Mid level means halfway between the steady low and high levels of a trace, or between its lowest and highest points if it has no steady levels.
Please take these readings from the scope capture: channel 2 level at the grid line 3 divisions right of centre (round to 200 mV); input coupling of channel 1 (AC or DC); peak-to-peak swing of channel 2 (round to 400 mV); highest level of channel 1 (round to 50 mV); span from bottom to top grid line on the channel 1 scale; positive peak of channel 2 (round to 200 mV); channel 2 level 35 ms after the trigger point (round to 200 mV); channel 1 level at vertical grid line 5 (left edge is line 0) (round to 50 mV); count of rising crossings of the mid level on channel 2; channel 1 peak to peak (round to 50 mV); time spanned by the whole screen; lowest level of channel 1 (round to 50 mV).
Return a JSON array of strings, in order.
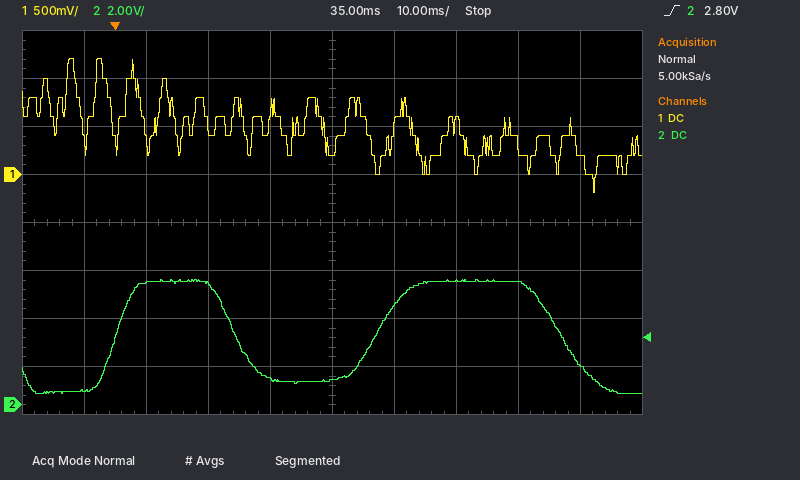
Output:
["5.2 V", "DC", "4.8 V", "1.20 V", "4 V", "5.2 V", "1.0 V", "200 mV", "2", "1.40 V", "100 ms", "-200 mV"]
